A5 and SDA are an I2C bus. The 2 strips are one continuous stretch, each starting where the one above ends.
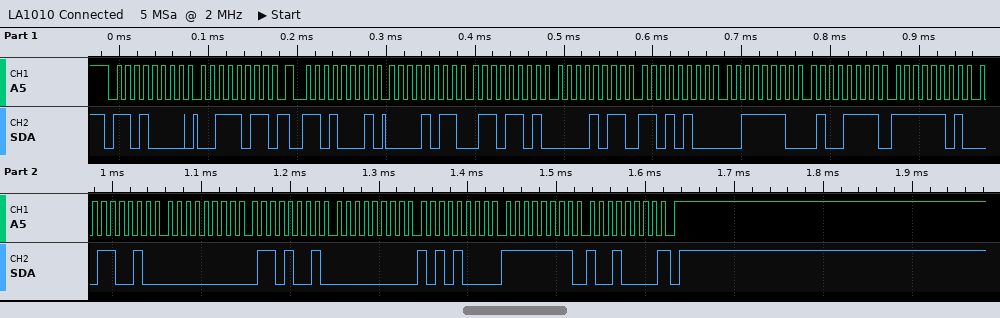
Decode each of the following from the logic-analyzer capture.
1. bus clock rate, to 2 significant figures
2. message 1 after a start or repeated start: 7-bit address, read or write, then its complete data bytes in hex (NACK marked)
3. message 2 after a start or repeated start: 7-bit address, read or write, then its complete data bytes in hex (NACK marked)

100 kHz
0x68 write: 3B
0x68 read: 0B 6D 0B D4 3E 4F FD 32 00 69 00 A8 FF 90 NACK
